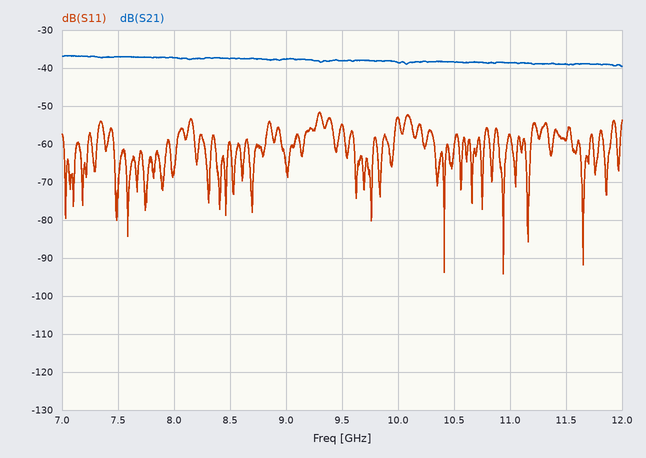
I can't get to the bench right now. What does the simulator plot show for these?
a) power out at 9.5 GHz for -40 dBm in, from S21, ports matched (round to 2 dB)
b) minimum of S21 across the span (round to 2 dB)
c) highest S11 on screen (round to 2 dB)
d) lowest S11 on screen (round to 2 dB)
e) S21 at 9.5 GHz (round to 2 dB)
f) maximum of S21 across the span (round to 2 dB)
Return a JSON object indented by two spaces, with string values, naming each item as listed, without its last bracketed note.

{
  "power out at 9.5 GHz for -40 dBm in, from S21, ports matched": "-78 dBm",
  "minimum of S21 across the span": "-40 dB",
  "highest S11 on screen": "-52 dB",
  "lowest S11 on screen": "-94 dB",
  "S21 at 9.5 GHz": "-38 dB",
  "maximum of S21 across the span": "-36 dB"
}
